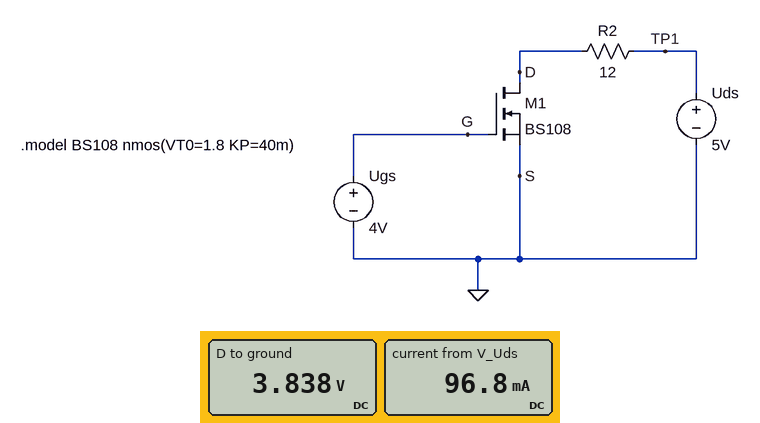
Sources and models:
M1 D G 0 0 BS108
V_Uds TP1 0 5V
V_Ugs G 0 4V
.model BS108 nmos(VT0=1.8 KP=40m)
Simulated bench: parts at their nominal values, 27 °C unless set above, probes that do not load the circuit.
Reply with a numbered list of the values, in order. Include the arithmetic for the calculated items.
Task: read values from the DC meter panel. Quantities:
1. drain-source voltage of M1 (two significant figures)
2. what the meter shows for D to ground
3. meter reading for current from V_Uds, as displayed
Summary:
1. 3.838 V = 3.8 V
2. 3.838 V
3. 96.8 mA
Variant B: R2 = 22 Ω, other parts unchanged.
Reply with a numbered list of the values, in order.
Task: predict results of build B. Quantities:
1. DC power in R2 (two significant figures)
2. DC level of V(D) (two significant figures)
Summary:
1. 210 mW
2. 2.9 V
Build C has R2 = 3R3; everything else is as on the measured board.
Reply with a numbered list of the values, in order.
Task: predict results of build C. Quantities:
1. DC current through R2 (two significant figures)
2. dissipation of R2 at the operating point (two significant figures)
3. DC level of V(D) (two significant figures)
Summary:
1. 97 mA
2. 31 mW
3. 4.7 V
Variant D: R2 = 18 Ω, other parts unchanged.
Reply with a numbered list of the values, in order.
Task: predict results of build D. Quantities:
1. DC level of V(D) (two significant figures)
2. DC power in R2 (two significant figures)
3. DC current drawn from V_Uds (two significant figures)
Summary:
1. 3.3 V
2. 170 mW
3. 97 mA
